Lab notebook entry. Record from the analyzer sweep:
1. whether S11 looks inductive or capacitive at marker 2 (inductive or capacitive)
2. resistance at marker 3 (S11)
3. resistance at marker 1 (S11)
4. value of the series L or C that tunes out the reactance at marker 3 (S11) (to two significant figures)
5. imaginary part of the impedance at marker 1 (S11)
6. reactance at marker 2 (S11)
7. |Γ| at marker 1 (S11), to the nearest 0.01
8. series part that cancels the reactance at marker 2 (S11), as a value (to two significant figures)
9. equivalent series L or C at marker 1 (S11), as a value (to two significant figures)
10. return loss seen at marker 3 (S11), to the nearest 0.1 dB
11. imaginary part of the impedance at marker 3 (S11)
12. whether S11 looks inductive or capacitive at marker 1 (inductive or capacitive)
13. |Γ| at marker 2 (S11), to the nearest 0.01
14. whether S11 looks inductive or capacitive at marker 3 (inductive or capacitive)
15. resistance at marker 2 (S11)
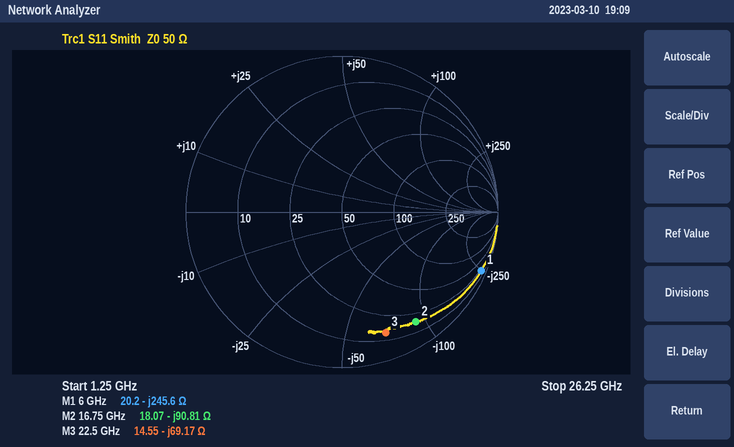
capacitive
14.55 Ω
20.2 Ω
490 pH
-245.6 Ω
-90.81 Ω
0.97
860 pH
110 fF
1.7 dB
-69.17 Ω
capacitive
0.85
capacitive
18.07 Ω
